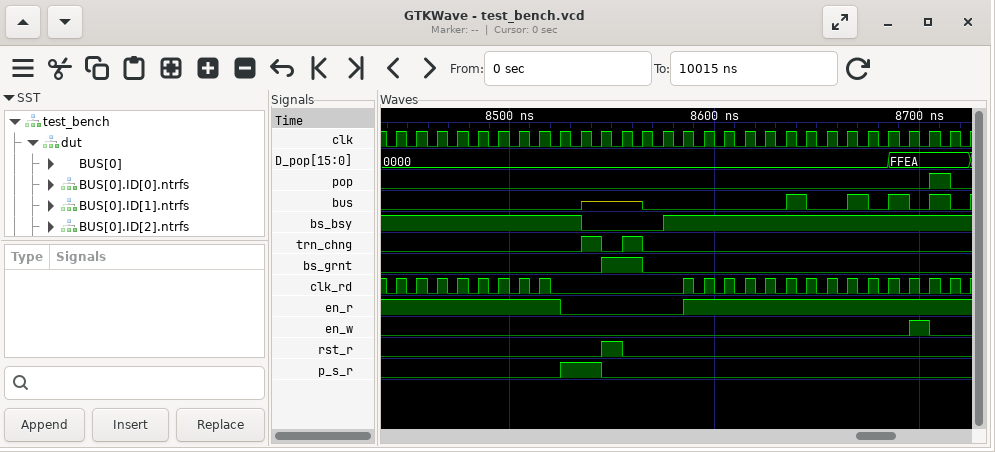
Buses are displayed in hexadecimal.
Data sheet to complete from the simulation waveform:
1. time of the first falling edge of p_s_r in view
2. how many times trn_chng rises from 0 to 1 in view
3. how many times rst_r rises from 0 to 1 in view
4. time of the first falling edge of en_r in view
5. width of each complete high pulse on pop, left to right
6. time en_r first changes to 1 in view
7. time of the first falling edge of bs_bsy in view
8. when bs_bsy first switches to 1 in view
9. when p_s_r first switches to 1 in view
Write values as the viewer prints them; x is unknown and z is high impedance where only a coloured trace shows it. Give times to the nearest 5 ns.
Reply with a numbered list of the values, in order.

1. 8545 ns
2. 2
3. 1
4. 8525 ns
5. 10 ns
6. 8585 ns
7. 8535 ns
8. 8575 ns
9. 8525 ns
